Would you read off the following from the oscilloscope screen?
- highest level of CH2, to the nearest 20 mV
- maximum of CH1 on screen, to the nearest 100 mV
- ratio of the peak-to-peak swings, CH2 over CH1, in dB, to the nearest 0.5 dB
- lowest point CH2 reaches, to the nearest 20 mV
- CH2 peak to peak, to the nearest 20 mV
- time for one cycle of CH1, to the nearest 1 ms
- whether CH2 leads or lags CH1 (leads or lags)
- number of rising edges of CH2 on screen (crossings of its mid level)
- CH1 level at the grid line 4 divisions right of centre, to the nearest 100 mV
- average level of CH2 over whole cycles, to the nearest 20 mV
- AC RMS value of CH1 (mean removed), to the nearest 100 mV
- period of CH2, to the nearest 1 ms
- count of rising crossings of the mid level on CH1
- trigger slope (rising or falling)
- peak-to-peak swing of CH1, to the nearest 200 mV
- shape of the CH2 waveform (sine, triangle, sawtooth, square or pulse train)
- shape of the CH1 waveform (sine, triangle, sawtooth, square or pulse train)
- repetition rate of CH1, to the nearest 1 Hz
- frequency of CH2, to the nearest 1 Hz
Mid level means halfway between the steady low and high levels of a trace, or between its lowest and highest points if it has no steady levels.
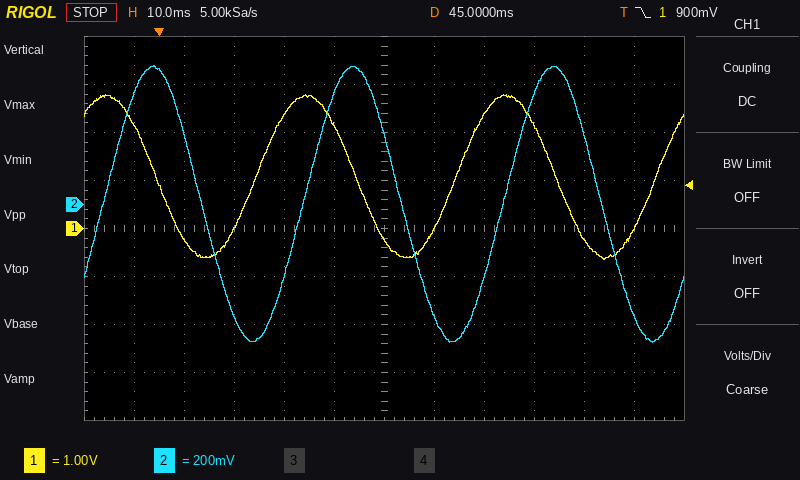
580 mV
2.8 V
-9.5 dB
-580 mV
1.16 V
40 ms
lags
3
-200 mV
0 mV
1.2 V
40 ms
3
falling
3.4 V
sine
sine
25 Hz
25 Hz
